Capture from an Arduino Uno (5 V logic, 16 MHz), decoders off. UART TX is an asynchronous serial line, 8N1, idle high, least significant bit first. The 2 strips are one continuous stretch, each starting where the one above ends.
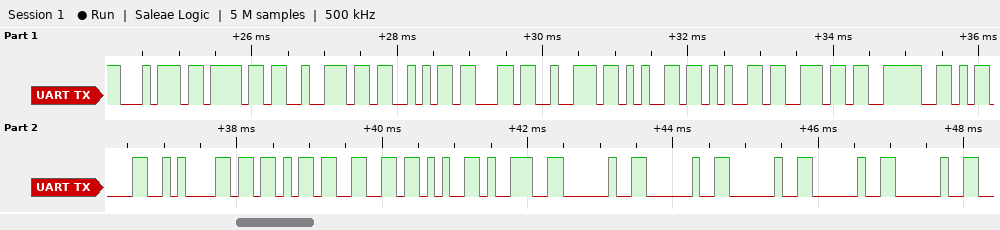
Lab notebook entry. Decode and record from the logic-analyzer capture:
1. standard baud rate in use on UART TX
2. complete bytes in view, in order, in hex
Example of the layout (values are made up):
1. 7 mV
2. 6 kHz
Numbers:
1. 9600 baud
2. 0x74 0x6F 0x72 0x53 0x63 0x72 0x65 0x65 0x6E 0x3E 0x0D 0x0A 0x5B 0x33 0x2B 0x39 0x20 0x20 0x20 0x20 0x20
